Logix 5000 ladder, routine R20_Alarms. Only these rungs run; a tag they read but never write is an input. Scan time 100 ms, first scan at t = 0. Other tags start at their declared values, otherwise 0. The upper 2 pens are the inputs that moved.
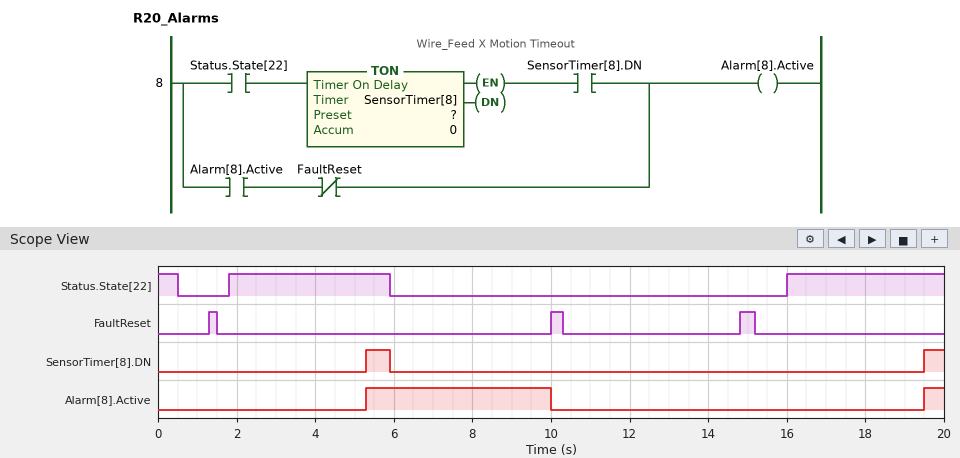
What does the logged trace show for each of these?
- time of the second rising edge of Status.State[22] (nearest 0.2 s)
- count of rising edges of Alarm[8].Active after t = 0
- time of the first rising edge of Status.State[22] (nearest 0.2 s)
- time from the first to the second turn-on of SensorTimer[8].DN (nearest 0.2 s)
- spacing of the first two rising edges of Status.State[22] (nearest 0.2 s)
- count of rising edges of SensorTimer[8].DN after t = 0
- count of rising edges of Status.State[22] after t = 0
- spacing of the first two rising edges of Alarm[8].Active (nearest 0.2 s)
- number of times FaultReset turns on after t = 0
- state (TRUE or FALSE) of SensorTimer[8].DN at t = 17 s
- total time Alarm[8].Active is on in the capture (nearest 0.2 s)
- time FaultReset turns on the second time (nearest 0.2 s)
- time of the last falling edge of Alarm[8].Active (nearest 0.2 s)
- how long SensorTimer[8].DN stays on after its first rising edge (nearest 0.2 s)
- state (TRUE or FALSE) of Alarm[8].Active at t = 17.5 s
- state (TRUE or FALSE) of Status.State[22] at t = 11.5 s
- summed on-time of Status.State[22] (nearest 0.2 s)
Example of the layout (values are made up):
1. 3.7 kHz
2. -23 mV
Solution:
1. 16.0 s
2. 2
3. 1.8 s
4. 14.2 s
5. 14.2 s
6. 2
7. 2
8. 14.2 s
9. 3
10. FALSE
11. 5.2 s
12. 10.0 s
13. 10.0 s
14. 0.6 s
15. FALSE
16. FALSE
17. 8.6 s
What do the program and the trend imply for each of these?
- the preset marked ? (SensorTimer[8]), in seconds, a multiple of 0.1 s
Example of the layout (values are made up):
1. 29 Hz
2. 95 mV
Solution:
1. 3.5 s
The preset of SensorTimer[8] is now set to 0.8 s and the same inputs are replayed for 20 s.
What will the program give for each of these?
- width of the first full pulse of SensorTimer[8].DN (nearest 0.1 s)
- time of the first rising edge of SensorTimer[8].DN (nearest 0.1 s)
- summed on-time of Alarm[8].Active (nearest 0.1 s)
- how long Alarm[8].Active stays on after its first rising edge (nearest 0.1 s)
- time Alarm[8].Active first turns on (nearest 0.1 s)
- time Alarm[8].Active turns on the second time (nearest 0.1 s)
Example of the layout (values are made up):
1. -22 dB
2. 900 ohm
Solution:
1. 3.3 s
2. 2.6 s
3. 10.6 s
4. 7.4 s
5. 2.6 s
6. 16.8 s
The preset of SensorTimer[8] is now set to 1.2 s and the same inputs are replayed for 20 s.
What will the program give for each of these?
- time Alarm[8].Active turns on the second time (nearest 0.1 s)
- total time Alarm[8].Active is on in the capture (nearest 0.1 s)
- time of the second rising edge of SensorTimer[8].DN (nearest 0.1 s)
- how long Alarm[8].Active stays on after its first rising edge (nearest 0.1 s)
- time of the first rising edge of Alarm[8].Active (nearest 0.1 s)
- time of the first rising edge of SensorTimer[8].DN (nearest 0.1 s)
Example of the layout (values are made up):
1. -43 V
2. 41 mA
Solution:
1. 17.2 s
2. 9.8 s
3. 17.2 s
4. 7.0 s
5. 3.0 s
6. 3.0 s
